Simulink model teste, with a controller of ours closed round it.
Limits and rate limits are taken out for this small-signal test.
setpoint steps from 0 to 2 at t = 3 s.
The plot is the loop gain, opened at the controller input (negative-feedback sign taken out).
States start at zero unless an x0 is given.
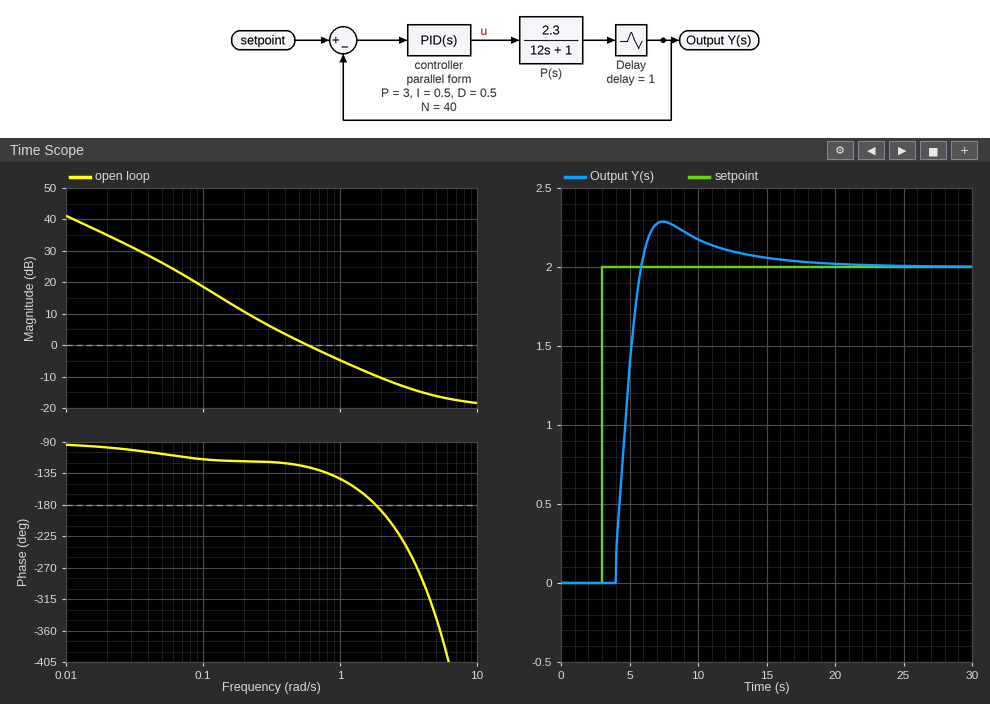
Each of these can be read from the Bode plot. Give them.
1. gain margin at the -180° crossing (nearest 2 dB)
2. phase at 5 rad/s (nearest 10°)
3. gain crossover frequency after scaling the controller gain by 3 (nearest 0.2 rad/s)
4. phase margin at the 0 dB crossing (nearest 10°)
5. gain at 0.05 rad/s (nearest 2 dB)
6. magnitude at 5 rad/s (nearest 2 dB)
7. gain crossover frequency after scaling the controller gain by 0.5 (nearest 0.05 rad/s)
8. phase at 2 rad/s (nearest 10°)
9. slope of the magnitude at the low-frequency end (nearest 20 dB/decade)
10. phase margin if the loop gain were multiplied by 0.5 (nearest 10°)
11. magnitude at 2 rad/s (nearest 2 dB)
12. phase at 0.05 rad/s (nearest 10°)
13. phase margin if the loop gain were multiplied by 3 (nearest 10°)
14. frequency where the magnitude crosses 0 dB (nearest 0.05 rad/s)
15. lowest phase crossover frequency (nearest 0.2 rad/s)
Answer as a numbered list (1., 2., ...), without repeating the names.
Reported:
1. 10 dB
2. -340°
3. 1.8 rad/s
4. 50°
5. 26 dB
6. -16 dB
7. 0.30 rad/s
8. -190°
9. -20 dB/decade
10. 60°
11. -10 dB
12. -110°
13. 0°
14. 0.60 rad/s
15. 1.8 rad/s
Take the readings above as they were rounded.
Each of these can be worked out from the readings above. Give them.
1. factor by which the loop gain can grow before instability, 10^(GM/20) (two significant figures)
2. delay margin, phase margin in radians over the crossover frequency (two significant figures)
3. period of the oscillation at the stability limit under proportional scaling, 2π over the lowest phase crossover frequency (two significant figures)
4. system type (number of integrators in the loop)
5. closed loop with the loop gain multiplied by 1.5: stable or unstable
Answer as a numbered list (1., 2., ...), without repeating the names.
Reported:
1. 3.2
2. 1.5 s
3. 3.5 s
4. 1
5. stable
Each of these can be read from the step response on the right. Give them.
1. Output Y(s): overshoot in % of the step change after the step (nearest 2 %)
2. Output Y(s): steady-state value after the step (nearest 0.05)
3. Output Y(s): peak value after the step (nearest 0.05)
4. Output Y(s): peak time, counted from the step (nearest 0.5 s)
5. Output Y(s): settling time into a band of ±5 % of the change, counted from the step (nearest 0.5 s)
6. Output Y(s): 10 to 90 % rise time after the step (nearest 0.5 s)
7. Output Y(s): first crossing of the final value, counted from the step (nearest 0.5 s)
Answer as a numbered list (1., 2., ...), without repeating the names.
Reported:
1. 14 %
2. 2.00
3. 2.30
4. 4.5 s
5. 9.5 s
6. 1.5 s
7. 3.0 s
